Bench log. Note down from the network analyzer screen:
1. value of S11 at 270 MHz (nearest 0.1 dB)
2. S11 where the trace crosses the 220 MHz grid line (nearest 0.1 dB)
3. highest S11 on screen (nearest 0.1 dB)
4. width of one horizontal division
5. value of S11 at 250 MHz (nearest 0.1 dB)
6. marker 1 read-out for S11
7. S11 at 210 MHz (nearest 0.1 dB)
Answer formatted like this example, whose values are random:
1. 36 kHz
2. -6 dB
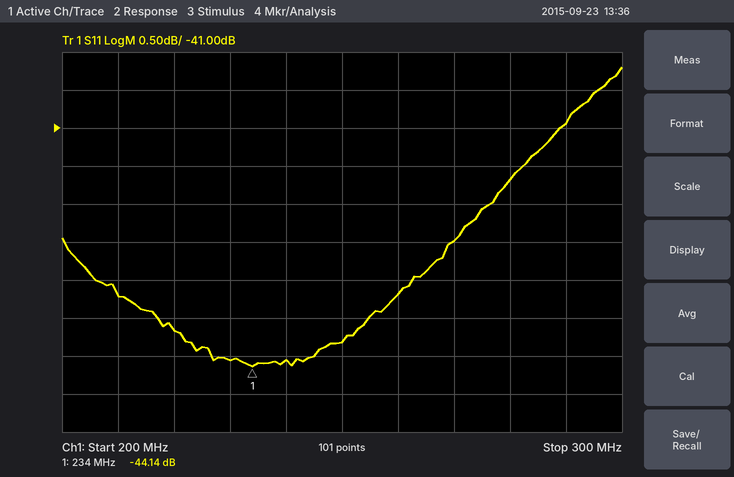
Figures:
1. -42.5 dB
2. -43.7 dB
3. -40.2 dB
4. 10 MHz
5. -43.8 dB
6. -44.14 dB
7. -43.2 dB
